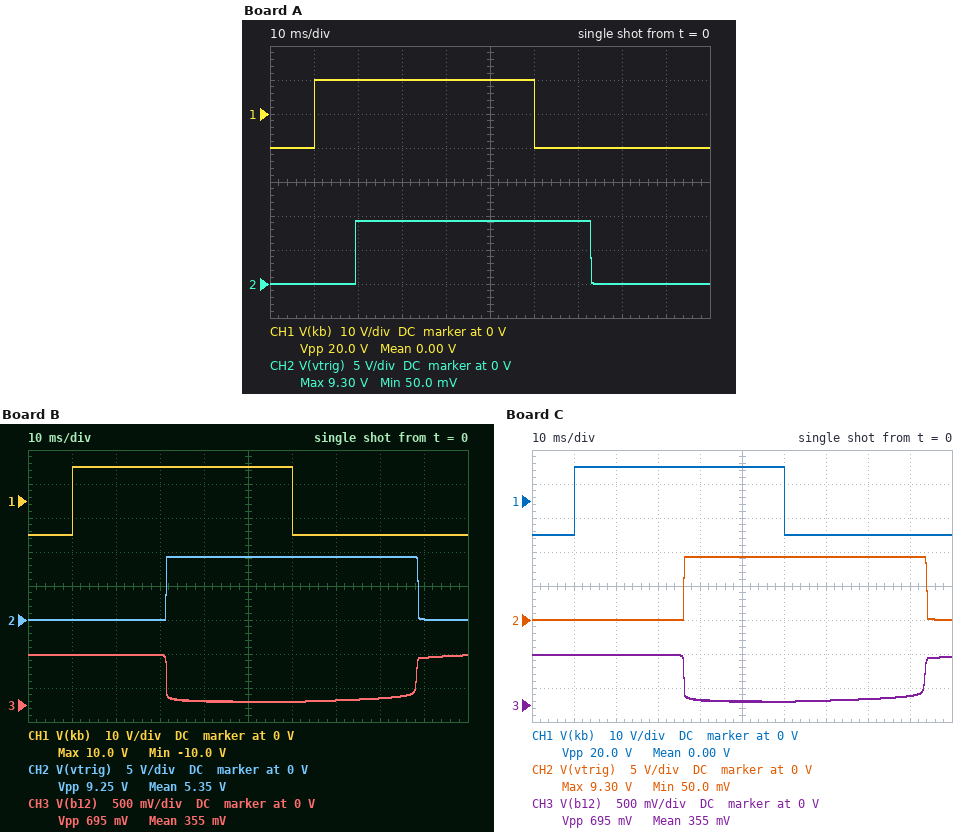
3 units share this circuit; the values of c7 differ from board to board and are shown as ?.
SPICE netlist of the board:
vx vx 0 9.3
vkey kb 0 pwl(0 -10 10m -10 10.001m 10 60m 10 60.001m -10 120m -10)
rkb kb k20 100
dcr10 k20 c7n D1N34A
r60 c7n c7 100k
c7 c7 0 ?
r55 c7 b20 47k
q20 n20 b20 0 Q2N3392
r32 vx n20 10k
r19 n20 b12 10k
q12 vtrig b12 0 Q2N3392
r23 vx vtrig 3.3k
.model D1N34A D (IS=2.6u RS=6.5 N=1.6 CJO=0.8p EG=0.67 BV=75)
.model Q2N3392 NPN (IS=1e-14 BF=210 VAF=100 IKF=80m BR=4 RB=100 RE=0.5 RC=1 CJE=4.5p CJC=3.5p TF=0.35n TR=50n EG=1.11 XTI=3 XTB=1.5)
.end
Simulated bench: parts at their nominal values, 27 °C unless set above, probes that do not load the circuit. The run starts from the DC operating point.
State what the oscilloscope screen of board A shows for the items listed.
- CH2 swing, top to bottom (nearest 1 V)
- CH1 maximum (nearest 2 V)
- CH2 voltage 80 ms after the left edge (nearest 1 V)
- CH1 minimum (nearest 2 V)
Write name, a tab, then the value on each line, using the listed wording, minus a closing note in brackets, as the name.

CH2 swing, top to bottom	9 V
CH1 maximum	10 V
CH2 voltage 80 ms after the left edge	0 V
CH1 minimum	-10 V
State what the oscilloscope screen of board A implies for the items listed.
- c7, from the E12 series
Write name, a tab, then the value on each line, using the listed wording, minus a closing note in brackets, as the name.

c7, from the E12 series	120 nF
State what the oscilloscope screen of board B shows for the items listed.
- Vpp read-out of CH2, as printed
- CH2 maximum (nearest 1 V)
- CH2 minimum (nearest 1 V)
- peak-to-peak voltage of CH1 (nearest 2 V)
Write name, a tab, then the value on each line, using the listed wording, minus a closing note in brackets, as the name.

Vpp read-out of CH2, as printed	9.25 V
CH2 maximum	9 V
CH2 minimum	0 V
peak-to-peak voltage of CH1	20 V
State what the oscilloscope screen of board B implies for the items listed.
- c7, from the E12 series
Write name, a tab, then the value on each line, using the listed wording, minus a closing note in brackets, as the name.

c7, from the E12 series	270 nF
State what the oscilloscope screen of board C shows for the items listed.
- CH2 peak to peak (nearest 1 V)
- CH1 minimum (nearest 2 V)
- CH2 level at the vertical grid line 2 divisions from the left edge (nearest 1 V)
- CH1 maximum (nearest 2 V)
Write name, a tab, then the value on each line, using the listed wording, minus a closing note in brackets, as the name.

CH2 peak to peak	9 V
CH1 minimum	-10 V
CH2 level at the vertical grid line 2 divisions from the left edge	0 V
CH1 maximum	10 V
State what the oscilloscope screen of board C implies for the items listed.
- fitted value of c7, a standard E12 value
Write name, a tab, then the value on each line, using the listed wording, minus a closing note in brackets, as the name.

fitted value of c7, a standard E12 value	330 nF
